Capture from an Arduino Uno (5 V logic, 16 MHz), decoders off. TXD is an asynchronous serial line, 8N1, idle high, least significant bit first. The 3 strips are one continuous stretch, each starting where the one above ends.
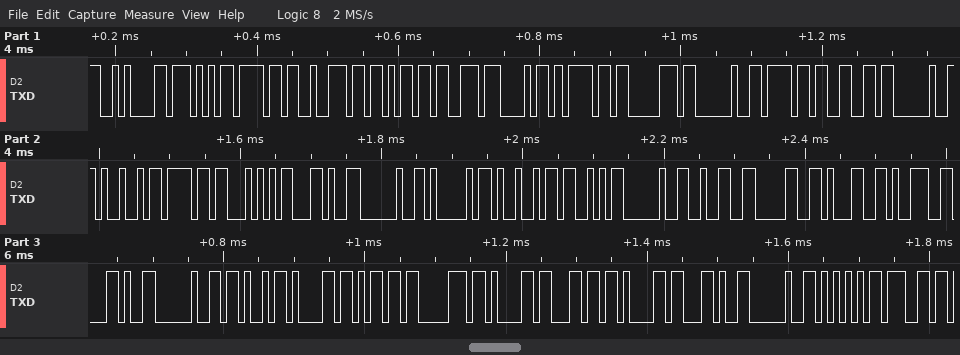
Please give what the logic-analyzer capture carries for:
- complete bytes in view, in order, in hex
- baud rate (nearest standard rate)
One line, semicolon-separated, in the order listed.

0A 57 6F 72 6B 73 68 6F 70 20 6F 66 20 49 6F 54 2C 20 41 49 53 20 32 30 31 39 2C 20 4B 61 6D 70 61 6C 61 2C 20 55 67; 115200 baud
